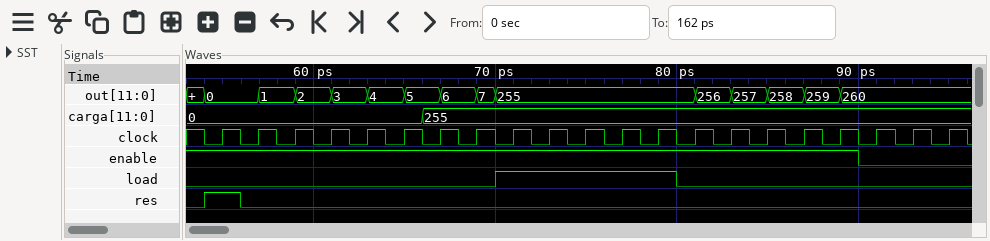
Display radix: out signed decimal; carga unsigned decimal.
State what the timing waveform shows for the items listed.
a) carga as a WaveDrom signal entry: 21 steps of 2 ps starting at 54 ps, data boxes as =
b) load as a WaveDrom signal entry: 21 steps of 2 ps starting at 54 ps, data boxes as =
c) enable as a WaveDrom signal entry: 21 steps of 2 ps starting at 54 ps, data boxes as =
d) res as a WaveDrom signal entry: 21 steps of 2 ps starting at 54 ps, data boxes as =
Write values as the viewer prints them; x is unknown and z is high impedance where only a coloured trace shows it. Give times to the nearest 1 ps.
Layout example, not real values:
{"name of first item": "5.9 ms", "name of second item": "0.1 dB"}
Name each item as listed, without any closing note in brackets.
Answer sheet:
{"carga as a WaveDrom signal entry: 21 steps of 2 ps starting at 54 ps, data boxes as =": "{name: 'carga', wave: '=.....=..............', data: '0 255'}", "load as a WaveDrom signal entry: 21 steps of 2 ps starting at 54 ps, data boxes as =": "{name: 'load', wave: '0.......1....0.......'}", "enable as a WaveDrom signal entry: 21 steps of 2 ps starting at 54 ps, data boxes as =": "{name: 'enable', wave: '1.................0..'}", "res as a WaveDrom signal entry: 21 steps of 2 ps starting at 54 ps, data boxes as =": "{name: 'res', wave: '10...................'}"}
